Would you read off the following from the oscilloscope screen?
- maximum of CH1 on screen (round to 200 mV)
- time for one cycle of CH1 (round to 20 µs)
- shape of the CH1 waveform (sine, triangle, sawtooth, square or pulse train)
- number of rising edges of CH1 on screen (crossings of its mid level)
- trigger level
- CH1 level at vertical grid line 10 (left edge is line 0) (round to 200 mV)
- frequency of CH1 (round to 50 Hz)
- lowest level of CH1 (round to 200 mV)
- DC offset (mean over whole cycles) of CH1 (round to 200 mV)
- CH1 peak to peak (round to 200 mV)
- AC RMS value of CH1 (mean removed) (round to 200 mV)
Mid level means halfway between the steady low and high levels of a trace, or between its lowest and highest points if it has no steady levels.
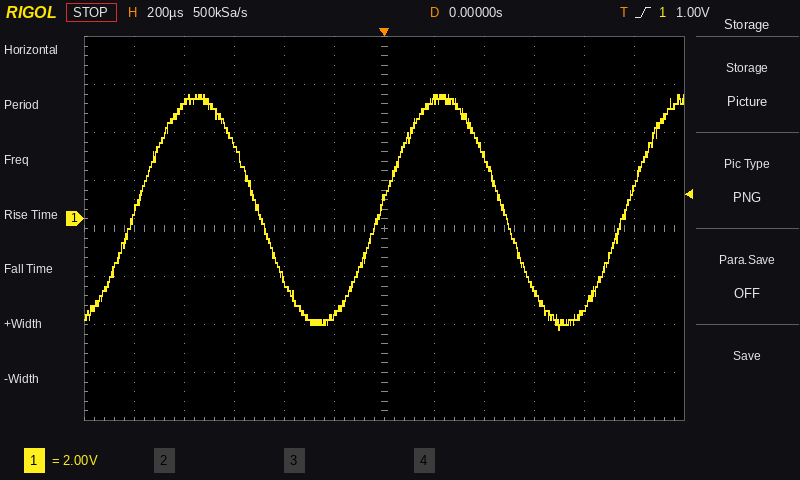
5.2 V
980 µs
sine
3
1.00 V
-3.8 V
1.00 kHz
-4.6 V
400 mV
9.8 V
3.4 V
